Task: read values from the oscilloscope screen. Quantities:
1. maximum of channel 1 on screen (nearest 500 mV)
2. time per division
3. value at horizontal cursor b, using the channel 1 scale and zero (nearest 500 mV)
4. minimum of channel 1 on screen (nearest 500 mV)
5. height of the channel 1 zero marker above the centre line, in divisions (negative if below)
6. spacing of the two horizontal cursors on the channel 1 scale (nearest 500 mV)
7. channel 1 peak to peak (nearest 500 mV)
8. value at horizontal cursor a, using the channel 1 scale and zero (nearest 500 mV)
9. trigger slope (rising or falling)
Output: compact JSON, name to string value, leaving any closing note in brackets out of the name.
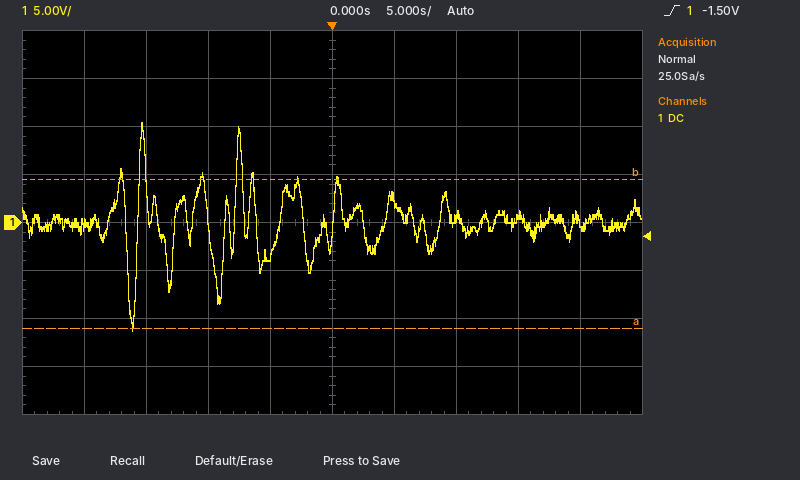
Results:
{"maximum of channel 1 on screen": "10.5 V", "time per division": "5 s", "value at horizontal cursor b, using the channel 1 scale and zero": "4.5 V", "minimum of channel 1 on screen": "-11.0 V", "height of the channel 1 zero marker above the centre line, in divisions": "0.0 div", "spacing of the two horizontal cursors on the channel 1 scale": "15.5 V", "channel 1 peak to peak": "21.5 V", "value at horizontal cursor a, using the channel 1 scale and zero": "-11.0 V", "trigger slope": "rising"}
